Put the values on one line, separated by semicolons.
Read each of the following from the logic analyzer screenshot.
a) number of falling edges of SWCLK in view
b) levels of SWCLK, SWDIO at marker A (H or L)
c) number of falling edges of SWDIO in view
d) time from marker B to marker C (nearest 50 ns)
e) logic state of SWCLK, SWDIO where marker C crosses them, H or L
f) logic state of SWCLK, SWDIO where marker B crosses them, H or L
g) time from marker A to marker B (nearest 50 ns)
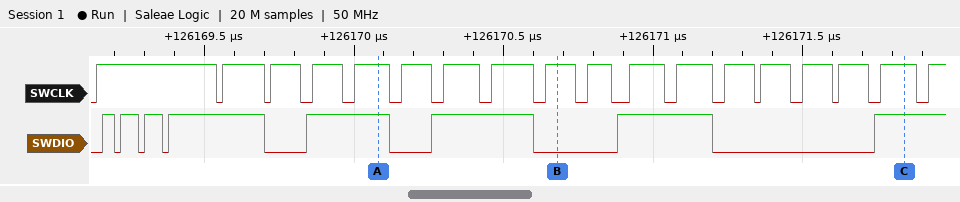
17; SWCLK=H, SWDIO=H; 7; 1150 ns; SWCLK=H, SWDIO=H; SWCLK=H, SWDIO=L; 600 ns
